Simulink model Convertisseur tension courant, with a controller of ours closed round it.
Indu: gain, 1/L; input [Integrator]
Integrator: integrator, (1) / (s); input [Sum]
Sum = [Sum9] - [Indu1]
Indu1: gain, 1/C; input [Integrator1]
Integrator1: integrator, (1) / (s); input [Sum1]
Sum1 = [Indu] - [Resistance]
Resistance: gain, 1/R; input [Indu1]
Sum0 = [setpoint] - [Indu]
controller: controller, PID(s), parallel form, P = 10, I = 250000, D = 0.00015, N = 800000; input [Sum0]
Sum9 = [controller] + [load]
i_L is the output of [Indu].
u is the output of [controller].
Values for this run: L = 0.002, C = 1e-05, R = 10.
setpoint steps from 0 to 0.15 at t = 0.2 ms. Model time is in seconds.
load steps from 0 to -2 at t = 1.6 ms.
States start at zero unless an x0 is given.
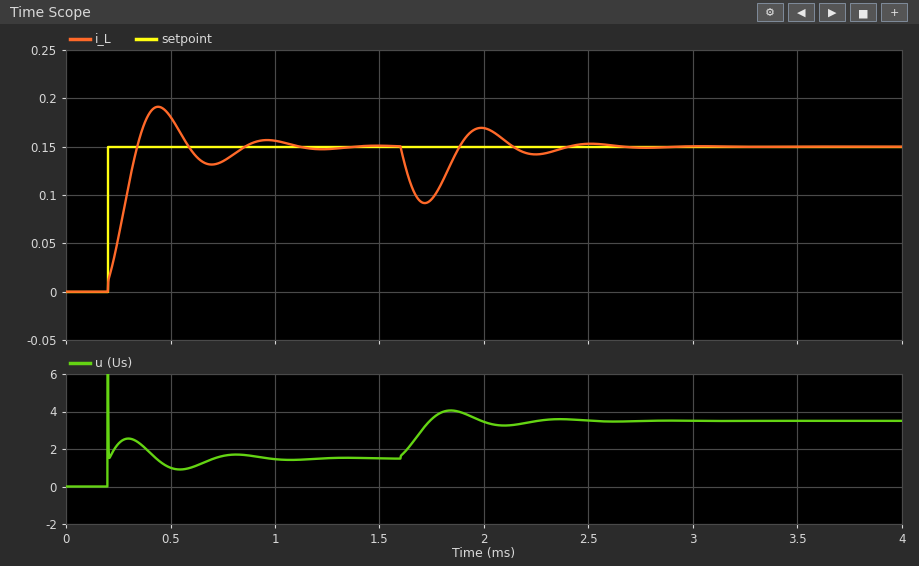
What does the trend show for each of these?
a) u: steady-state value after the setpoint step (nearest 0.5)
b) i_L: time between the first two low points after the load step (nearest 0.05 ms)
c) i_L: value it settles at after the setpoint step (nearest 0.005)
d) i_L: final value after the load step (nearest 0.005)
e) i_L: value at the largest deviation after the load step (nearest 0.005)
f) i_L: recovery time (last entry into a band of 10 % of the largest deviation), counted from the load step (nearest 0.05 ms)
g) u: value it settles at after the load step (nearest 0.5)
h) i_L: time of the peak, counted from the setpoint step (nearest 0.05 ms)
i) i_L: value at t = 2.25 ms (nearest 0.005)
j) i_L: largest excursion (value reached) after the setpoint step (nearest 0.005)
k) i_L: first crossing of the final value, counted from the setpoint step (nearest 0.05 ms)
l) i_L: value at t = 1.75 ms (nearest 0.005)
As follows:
1.5
0.55 ms
0.150
0.150
0.090
0.70 ms
3.5
0.25 ms
0.140
0.190
0.15 ms
0.095
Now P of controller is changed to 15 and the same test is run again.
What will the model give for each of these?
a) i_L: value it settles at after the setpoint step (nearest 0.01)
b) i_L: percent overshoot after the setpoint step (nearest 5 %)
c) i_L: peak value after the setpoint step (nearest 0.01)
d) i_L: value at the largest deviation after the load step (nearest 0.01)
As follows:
0.15
20 %
0.18
0.10
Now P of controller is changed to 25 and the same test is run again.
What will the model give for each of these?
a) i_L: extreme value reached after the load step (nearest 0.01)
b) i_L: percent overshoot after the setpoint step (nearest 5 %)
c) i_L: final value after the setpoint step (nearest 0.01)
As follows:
0.11
10 %
0.15
